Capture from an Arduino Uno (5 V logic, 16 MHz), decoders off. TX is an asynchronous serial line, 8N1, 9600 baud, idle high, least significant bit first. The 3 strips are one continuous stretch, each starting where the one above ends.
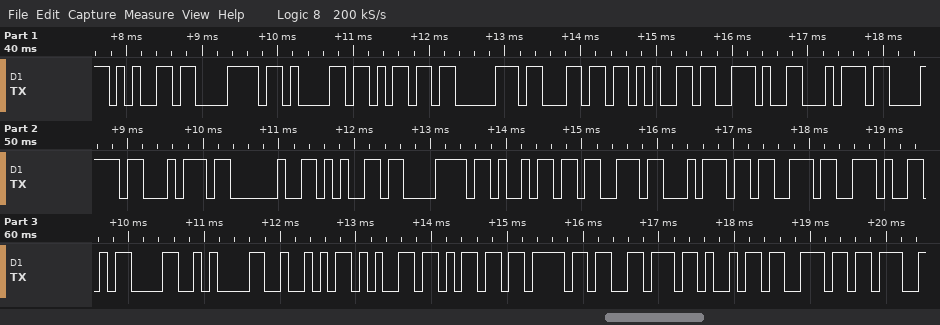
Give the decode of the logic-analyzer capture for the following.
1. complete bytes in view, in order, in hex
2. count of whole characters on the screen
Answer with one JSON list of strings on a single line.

["0x65 0x78 0x61 0x6D 0x70 0x6C 0x65 0x2E 0x74 0x78 0x74 0x20 0x65 0x78 0x69 0x73 0x74 0x73 0x2E 0x0D 0x0A 0x52 0x65 0x6D 0x6F 0x76 0x69 0x6E", "28"]
